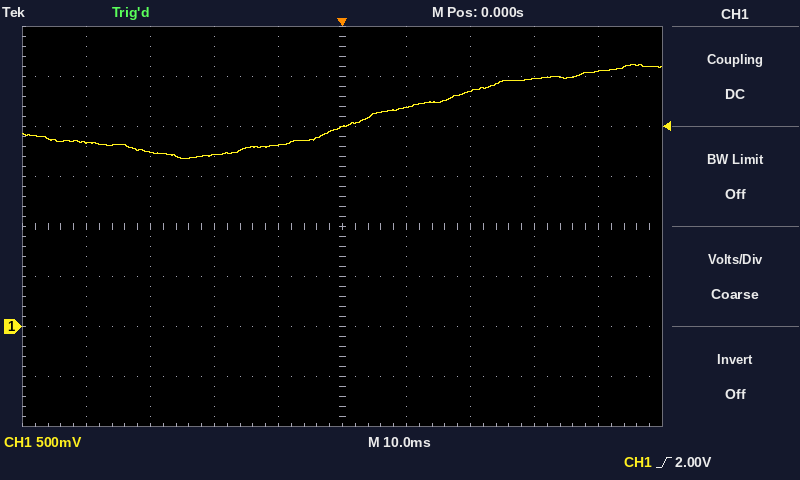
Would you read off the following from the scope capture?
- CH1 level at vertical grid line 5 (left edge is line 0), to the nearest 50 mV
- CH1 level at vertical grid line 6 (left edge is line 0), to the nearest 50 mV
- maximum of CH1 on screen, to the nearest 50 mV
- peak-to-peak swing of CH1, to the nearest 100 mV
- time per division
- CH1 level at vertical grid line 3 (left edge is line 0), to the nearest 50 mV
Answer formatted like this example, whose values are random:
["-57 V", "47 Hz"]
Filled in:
["2.00 V", "2.20 V", "2.60 V", "900 mV", "10 ms", "1.70 V"]
